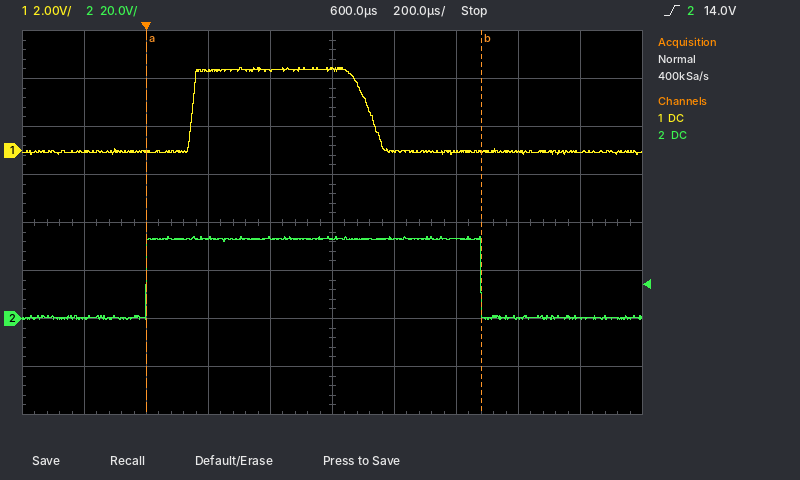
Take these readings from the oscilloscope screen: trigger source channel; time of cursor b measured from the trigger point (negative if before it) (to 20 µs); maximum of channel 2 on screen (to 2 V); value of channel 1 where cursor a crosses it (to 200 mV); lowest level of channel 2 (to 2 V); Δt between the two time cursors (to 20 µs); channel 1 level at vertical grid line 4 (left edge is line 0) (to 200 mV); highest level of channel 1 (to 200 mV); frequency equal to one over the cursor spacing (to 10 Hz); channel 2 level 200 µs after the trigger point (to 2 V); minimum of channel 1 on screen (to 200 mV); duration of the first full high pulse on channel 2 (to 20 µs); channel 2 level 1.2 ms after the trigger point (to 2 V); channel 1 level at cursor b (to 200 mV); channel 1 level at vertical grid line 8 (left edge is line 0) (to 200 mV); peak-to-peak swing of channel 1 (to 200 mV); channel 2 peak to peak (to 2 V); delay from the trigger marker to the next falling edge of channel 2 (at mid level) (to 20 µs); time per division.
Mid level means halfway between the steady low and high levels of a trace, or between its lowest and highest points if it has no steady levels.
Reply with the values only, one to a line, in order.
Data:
channel 2
+1.08 ms
34 V
0.0 V
0 V
1.08 ms
3.4 V
3.4 V
930 Hz
34 V
-200 mV
1.08 ms
0 V
0.0 V
0.0 V
3.6 V
34 V
1.08 ms
200 µs
